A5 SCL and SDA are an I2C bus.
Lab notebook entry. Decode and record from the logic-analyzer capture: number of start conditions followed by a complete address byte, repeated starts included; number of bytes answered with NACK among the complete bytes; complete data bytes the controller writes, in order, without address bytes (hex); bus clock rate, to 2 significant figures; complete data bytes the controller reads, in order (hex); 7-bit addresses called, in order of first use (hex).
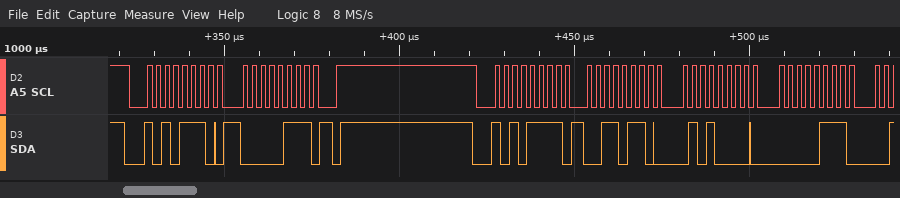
2
0
07
400 kHz
36 50 07
0x57
